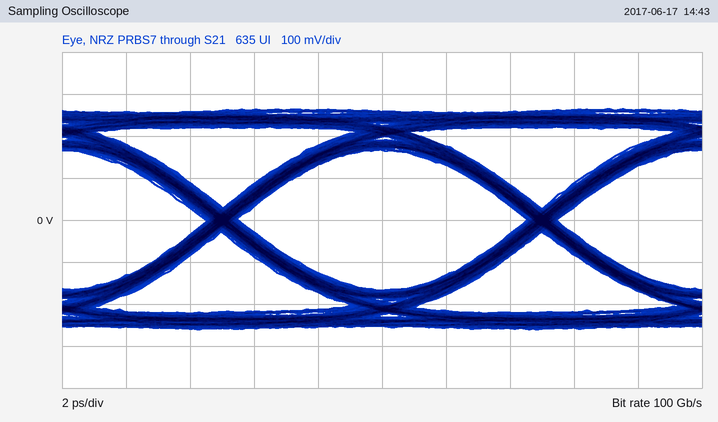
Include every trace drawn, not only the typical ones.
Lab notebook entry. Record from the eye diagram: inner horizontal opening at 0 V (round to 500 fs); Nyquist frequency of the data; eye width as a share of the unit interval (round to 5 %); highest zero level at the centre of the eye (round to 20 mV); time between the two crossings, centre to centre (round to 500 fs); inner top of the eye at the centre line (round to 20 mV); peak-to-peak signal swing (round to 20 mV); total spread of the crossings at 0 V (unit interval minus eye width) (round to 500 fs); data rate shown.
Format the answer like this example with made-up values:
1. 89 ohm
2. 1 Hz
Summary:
1. 9.0 ps
2. 50 GHz
3. 90 %
4. -160 mV
5. 10.0 ps
6. 160 mV
7. 520 mV
8. 1.0 ps
9. 100 Gb/s
